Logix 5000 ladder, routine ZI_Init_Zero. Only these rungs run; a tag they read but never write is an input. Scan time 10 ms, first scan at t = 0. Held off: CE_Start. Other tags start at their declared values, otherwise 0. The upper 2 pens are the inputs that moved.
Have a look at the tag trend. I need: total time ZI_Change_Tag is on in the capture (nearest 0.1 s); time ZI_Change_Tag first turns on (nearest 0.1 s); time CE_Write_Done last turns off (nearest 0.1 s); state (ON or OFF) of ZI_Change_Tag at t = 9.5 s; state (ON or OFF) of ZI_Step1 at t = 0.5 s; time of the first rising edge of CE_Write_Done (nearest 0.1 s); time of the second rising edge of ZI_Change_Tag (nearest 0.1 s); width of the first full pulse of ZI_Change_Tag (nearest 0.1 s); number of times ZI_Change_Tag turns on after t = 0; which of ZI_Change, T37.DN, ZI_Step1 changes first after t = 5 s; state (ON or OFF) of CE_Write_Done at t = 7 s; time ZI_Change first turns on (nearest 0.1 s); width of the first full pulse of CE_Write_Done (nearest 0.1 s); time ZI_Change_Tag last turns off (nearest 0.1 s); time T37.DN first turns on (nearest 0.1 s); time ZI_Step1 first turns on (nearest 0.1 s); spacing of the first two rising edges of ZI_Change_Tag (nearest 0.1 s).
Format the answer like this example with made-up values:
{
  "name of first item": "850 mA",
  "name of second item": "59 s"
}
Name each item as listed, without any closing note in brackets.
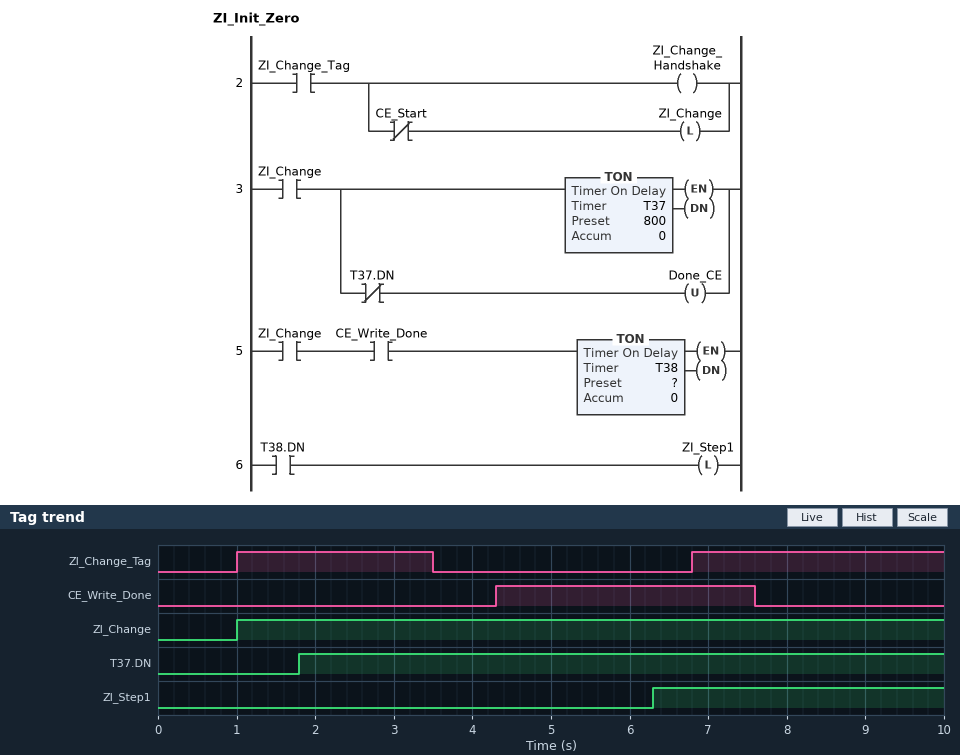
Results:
{
  "total time ZI_Change_Tag is on in the capture": "5.7 s",
  "time ZI_Change_Tag first turns on": "1.0 s",
  "time CE_Write_Done last turns off": "7.6 s",
  "state (ON or OFF) of ZI_Change_Tag at t = 9.5 s": "ON",
  "state (ON or OFF) of ZI_Step1 at t = 0.5 s": "OFF",
  "time of the first rising edge of CE_Write_Done": "4.3 s",
  "time of the second rising edge of ZI_Change_Tag": "6.8 s",
  "width of the first full pulse of ZI_Change_Tag": "2.5 s",
  "number of times ZI_Change_Tag turns on after t = 0": "2",
  "which of ZI_Change, T37.DN, ZI_Step1 changes first after t = 5 s": "ZI_Step1",
  "state (ON or OFF) of CE_Write_Done at t = 7 s": "ON",
  "time ZI_Change first turns on": "1.0 s",
  "width of the first full pulse of CE_Write_Done": "3.3 s",
  "time ZI_Change_Tag last turns off": "3.5 s",
  "time T37.DN first turns on": "1.8 s",
  "time ZI_Step1 first turns on": "6.3 s",
  "spacing of the first two rising edges of ZI_Change_Tag": "5.8 s"
}
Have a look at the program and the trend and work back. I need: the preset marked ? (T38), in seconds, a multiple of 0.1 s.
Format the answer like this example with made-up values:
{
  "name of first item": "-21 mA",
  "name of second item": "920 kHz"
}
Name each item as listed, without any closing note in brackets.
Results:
{
  "the preset marked ? (T38), in seconds, a multiple of 0.1 s": "2.0 s"
}
